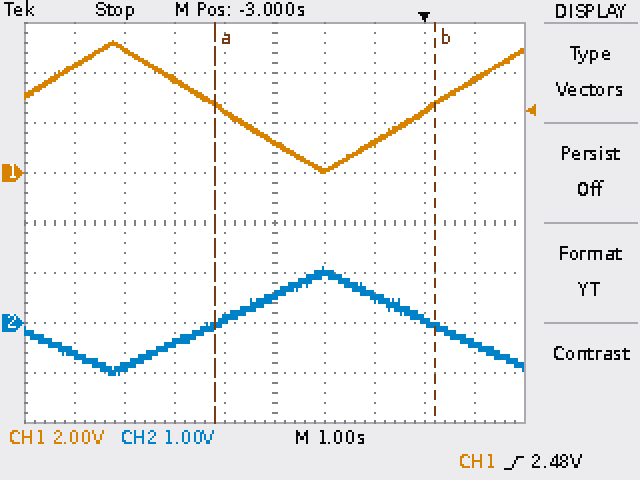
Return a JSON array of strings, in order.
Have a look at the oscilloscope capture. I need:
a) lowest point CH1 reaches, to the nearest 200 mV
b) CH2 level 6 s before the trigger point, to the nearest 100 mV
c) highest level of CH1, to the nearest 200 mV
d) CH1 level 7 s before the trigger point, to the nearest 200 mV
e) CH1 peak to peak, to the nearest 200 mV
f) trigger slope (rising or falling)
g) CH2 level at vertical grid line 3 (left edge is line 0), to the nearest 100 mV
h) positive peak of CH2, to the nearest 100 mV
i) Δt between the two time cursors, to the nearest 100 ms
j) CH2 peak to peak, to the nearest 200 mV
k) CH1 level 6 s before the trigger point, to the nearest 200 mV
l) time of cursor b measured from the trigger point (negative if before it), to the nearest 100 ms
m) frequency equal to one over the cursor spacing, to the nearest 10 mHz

["0.0 V", "-900 mV", "5.2 V", "4.2 V", "5.2 V", "rising", "-400 mV", "1.1 V", "4.4 s", "2.2 V", "5.0 V", "+200 ms", "230 mHz"]
